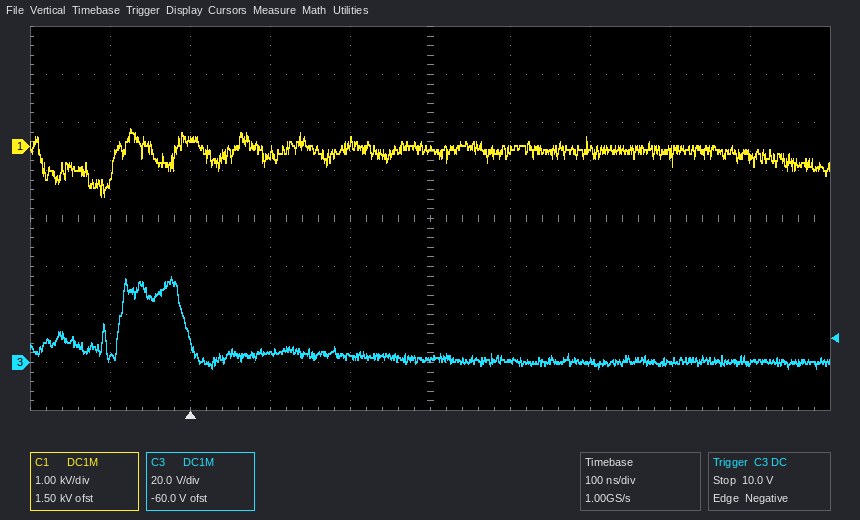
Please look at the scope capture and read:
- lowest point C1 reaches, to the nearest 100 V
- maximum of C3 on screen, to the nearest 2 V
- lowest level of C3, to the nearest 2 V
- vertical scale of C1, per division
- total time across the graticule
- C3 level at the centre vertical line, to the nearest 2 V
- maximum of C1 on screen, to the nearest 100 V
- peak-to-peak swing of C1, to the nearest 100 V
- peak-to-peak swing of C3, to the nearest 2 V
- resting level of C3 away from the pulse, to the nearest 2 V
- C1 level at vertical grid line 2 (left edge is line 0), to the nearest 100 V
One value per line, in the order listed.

-1.0 kV
36 V
-2 V
1 kV
1 µs
2 V
400 V
1.4 kV
38 V
0 V
100 V
